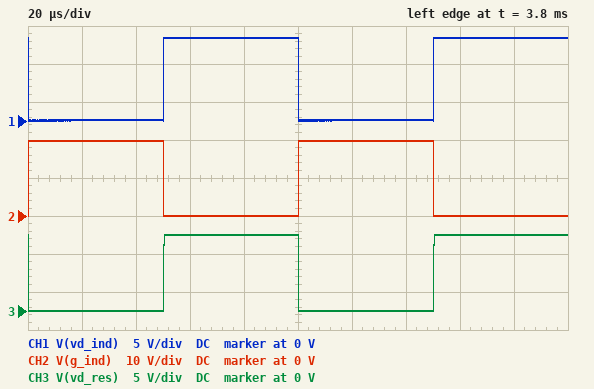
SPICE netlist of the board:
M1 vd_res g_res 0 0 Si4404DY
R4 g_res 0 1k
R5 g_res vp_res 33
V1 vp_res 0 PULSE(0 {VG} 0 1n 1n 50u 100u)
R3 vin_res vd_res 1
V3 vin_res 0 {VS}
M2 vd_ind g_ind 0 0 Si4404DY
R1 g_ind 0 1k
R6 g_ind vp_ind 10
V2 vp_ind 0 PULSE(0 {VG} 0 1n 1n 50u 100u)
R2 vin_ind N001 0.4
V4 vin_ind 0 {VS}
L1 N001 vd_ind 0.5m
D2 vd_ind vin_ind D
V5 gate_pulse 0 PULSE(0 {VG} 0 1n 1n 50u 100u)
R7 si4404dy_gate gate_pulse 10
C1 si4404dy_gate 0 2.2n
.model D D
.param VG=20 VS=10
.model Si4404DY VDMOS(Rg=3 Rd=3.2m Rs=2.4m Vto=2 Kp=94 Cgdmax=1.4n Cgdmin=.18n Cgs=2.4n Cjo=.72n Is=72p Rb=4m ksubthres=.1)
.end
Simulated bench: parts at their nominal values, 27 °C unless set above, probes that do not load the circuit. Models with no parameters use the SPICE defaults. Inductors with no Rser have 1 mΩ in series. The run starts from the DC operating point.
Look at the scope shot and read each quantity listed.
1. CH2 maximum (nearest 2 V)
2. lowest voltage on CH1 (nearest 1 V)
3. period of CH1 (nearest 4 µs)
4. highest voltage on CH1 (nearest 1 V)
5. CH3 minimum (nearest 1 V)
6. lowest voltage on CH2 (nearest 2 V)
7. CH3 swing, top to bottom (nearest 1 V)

20 V
0 V
100 µs
11 V
0 V
0 V
10 V
